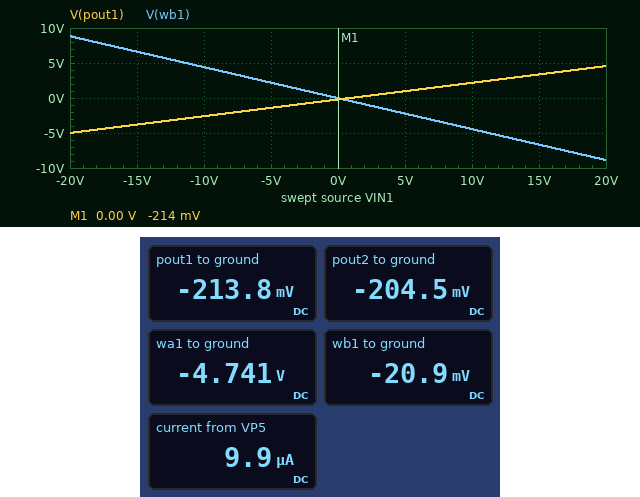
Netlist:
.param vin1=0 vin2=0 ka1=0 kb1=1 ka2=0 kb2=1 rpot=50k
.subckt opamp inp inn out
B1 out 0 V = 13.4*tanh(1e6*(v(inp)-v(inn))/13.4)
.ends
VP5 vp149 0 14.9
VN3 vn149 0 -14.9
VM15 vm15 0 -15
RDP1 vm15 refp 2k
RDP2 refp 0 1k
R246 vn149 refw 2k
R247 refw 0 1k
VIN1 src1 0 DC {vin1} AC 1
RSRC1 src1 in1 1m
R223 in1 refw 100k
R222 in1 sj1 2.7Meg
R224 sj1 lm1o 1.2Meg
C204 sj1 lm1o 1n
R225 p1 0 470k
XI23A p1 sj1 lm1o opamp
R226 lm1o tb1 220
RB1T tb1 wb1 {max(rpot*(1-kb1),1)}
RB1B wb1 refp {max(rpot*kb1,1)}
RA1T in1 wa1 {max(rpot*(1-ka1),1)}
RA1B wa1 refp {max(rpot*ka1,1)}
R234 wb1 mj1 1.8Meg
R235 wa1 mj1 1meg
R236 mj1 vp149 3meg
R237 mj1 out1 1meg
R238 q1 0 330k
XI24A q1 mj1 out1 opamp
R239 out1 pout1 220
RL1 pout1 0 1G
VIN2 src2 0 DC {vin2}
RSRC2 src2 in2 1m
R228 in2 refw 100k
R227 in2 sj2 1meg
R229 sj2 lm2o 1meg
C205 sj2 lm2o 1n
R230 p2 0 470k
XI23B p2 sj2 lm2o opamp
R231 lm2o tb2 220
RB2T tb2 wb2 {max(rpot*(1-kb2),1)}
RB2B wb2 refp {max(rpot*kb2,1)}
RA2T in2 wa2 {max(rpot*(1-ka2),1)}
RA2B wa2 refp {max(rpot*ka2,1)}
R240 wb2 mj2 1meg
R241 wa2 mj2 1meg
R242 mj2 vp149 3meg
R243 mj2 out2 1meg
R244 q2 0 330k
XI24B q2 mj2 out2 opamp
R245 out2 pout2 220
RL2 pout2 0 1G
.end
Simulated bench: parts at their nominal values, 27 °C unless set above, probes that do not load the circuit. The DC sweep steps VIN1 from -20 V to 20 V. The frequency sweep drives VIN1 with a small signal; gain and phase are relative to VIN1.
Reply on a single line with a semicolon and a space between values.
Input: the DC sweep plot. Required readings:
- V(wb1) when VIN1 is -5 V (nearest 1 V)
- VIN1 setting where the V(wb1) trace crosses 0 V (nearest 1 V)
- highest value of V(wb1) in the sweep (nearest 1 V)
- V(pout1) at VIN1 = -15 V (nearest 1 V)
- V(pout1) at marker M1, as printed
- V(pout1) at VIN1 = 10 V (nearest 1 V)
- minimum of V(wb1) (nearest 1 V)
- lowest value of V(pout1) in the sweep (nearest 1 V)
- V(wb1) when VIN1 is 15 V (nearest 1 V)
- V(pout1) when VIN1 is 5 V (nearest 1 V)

2 V; 0 V; 9 V; -4 V; -214 mV; 2 V; -9 V; -5 V; -7 V; 1 V
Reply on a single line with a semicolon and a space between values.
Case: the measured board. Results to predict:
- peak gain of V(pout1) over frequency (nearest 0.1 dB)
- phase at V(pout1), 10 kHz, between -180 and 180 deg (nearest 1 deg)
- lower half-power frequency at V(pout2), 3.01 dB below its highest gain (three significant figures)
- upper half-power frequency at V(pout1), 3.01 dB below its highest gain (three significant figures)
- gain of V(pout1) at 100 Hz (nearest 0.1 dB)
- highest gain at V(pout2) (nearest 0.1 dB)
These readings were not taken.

-12.4 dB; -165 deg; 81.6 Hz; 133 Hz; -14.4 dB; -37.9 dB
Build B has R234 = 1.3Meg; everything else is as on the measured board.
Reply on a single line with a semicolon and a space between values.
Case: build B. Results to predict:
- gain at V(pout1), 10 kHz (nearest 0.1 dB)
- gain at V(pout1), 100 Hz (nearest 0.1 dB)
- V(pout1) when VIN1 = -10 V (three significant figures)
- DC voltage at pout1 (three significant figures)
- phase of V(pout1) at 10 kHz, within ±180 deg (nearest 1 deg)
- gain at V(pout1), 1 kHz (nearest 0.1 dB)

-37.4 dB; -11.5 dB; -3.54 V; -209 mV; -160 deg; -26.8 dB
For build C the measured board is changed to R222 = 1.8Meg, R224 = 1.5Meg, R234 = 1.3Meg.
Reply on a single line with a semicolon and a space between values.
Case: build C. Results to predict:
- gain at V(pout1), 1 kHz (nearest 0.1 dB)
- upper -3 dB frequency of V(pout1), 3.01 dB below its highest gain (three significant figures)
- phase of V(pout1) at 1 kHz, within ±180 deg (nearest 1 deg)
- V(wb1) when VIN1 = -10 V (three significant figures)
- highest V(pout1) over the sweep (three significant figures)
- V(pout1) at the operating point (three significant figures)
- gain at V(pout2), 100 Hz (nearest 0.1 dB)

-23.3 dB; 106 Hz; -95 deg; 8.27 V; 10.0 V; -209 mV; -41.1 dB
